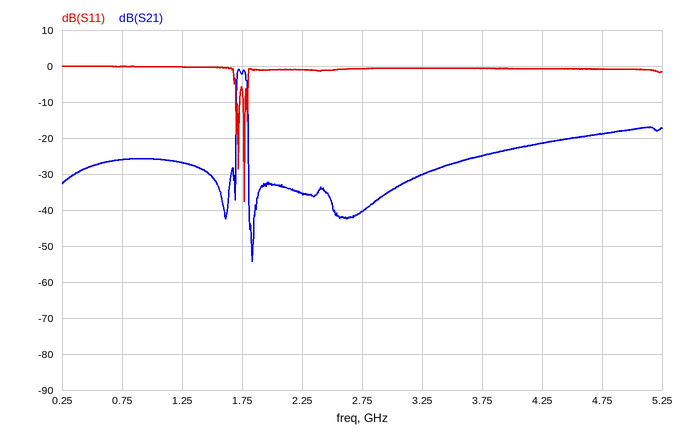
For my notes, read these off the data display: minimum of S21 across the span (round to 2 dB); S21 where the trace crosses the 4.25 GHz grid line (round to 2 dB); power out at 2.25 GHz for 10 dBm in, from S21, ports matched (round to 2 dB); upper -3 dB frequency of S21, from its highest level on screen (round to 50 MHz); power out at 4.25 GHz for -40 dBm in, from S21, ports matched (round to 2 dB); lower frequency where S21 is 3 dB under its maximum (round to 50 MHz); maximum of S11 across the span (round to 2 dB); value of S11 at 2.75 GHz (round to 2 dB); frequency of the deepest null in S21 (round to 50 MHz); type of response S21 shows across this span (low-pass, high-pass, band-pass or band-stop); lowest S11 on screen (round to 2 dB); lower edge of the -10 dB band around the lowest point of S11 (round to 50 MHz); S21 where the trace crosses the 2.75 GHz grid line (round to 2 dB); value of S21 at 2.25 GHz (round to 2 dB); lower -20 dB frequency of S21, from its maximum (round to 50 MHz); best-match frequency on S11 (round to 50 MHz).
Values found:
-54 dB
-22 dB
-26 dBm
1.80 GHz
-62 dBm
1.70 GHz
0 dB
0 dB
1.85 GHz
band-pass
-38 dB
1.75 GHz
-40 dB
-36 dB
1.70 GHz
1.75 GHz
